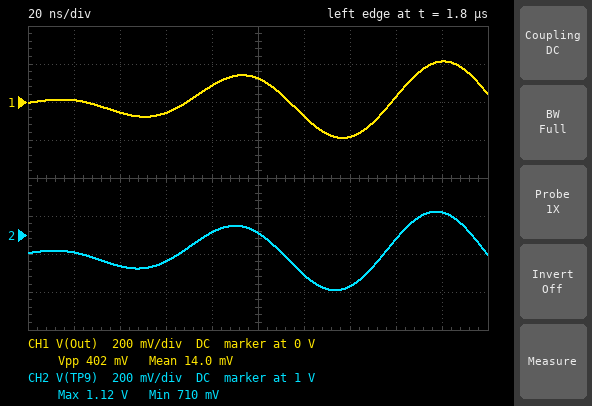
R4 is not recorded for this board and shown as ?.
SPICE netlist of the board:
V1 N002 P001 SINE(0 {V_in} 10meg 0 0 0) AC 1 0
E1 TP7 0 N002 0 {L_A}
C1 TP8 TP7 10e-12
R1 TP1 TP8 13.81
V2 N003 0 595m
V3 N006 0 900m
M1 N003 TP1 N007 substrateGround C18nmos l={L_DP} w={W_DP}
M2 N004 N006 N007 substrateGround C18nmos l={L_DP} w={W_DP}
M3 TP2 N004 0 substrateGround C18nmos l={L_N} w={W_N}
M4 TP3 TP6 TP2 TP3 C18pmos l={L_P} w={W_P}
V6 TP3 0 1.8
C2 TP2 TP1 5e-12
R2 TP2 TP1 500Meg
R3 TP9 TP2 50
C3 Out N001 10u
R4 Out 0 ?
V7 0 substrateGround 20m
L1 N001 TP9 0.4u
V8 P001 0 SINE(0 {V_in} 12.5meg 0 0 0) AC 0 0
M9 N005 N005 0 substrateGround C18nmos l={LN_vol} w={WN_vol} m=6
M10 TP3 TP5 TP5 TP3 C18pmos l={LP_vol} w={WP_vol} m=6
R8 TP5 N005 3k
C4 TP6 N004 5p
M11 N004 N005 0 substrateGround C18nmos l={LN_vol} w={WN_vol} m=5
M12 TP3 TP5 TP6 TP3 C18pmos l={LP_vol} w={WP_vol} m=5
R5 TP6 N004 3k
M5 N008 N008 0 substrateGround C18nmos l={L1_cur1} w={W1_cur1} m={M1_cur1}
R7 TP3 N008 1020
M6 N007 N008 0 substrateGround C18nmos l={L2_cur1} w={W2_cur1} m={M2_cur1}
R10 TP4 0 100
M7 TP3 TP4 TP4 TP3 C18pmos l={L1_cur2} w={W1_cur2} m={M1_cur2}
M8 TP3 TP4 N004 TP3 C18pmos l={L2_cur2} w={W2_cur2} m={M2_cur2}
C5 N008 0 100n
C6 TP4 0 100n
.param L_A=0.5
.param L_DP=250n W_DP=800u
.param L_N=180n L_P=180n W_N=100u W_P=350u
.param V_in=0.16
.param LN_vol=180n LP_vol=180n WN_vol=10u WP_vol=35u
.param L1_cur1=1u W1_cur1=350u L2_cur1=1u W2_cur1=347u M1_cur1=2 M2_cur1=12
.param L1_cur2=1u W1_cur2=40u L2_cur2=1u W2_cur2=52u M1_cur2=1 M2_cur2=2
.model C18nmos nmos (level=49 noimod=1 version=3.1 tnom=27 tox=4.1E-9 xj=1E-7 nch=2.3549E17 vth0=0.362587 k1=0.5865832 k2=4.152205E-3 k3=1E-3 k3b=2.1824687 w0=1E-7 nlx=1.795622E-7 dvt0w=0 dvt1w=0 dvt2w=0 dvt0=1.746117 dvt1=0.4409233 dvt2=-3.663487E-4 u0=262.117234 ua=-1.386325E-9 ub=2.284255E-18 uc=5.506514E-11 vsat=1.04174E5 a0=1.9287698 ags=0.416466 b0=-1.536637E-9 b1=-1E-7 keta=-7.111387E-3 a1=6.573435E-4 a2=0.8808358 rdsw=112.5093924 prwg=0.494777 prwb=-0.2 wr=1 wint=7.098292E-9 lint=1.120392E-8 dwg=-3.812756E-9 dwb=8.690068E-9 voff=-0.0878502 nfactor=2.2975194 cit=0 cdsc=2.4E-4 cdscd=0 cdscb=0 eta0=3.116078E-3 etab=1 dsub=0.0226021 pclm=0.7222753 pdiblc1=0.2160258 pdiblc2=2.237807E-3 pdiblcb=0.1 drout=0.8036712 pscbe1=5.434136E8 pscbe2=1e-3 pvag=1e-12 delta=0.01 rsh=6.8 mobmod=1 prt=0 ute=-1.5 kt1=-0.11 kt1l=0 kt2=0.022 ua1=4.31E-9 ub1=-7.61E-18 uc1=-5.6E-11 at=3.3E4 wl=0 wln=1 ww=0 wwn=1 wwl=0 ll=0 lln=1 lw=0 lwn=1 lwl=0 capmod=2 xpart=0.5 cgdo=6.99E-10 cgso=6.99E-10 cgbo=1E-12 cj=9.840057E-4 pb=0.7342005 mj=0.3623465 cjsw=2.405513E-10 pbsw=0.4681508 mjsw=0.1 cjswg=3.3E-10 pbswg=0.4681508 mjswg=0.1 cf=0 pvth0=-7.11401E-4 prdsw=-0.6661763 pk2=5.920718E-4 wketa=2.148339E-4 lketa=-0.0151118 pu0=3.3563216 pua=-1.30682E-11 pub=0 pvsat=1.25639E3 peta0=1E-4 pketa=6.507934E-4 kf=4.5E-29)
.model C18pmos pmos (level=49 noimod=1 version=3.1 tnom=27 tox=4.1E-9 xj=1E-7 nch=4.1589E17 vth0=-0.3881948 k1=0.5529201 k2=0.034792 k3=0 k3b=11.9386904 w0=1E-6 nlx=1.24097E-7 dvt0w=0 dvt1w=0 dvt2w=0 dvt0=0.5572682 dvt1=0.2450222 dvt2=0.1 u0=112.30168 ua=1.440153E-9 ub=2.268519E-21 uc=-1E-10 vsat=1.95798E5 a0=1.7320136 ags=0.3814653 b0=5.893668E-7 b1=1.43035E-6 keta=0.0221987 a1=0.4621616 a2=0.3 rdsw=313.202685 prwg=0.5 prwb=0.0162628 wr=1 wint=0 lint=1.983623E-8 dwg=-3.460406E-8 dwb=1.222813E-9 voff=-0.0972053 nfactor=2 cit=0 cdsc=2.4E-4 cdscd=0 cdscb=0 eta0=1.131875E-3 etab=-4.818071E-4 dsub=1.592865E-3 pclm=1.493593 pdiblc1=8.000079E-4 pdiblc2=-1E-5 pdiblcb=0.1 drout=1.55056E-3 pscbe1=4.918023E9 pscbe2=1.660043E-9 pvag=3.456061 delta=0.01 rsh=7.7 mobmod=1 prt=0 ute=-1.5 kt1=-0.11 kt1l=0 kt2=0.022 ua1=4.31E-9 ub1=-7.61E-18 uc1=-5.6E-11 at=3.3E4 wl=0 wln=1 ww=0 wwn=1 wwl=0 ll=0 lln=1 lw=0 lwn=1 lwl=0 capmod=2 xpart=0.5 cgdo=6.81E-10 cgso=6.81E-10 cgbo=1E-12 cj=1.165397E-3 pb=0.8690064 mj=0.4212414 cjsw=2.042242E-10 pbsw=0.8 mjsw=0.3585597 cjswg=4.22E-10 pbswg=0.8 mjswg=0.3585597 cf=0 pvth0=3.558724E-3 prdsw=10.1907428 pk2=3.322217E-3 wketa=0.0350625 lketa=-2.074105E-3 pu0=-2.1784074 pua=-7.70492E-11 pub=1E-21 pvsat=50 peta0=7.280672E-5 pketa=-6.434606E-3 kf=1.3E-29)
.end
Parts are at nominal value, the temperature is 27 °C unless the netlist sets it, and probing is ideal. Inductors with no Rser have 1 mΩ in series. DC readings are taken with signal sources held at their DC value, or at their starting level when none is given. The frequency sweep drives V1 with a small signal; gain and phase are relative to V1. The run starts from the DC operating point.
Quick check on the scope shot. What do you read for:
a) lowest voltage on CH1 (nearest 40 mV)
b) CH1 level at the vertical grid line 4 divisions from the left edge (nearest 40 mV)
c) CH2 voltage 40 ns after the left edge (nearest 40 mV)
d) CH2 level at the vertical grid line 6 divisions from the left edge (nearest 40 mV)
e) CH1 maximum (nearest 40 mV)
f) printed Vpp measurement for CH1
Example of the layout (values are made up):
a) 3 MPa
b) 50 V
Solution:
a) -200 mV
b) 80 mV
c) 840 mV
d) 800 mV
e) 200 mV
f) 402 mV
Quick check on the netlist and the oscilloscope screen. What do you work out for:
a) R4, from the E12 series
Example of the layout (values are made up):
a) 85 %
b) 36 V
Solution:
a) 120 Ω
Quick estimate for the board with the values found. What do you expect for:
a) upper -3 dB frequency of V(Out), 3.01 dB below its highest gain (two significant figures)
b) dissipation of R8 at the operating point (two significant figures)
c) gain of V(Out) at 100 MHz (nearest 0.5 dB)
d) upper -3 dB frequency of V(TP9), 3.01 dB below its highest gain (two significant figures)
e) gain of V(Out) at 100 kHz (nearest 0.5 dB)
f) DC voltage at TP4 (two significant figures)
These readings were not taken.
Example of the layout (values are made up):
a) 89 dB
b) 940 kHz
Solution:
a) 68 MHz
b) 170 µW
c) -8.0 dB
d) 880 MHz
e) -3.0 dB
f) 140 mV
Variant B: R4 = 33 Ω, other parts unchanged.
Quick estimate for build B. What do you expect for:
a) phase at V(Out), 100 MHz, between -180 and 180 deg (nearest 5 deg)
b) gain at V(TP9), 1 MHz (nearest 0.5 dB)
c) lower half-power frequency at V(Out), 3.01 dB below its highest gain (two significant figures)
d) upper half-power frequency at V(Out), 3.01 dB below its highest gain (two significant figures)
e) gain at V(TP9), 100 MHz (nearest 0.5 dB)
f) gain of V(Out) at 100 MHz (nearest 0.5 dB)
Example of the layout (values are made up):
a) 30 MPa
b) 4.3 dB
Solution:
a) 100 deg
b) -8.5 dB
c) 200 Hz
d) 33 MHz
e) -0.5 dB
f) -18.0 dB
